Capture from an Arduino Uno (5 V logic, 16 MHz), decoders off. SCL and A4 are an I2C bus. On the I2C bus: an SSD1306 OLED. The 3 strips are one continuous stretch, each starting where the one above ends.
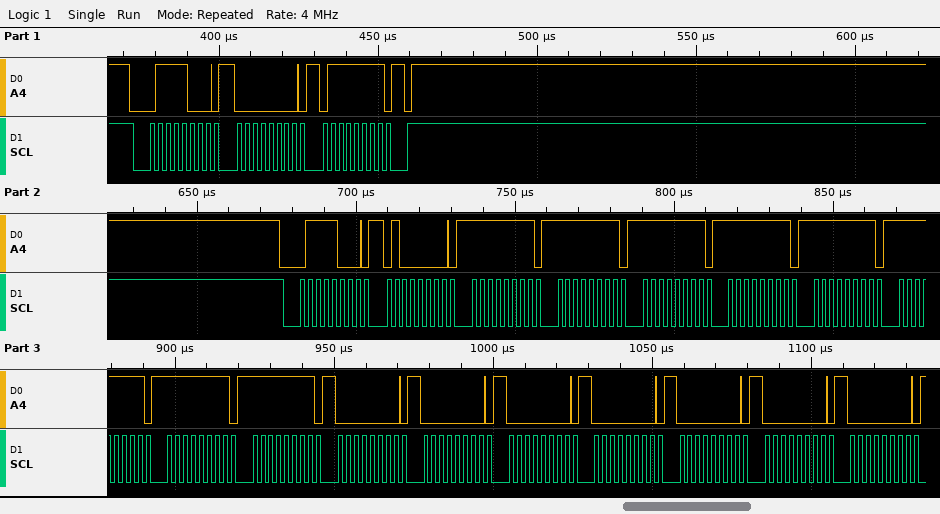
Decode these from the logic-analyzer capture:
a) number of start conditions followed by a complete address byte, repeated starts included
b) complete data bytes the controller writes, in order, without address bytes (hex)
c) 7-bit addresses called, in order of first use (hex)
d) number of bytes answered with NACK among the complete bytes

2
00 7F 40 FF FF FF FF FF FF FF FF 00 00 00 00 00 00 00
0x3C
0
